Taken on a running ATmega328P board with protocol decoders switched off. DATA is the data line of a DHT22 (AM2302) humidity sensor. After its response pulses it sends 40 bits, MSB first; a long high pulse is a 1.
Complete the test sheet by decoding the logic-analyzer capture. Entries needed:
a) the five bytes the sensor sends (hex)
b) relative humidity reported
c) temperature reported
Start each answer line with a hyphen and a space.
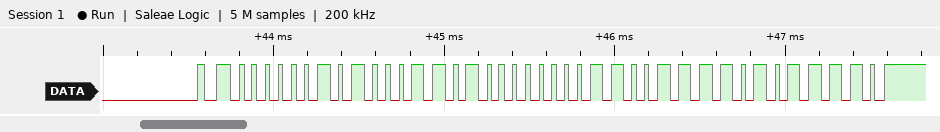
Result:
- 02 8D 00 CF 5E
- 65.3 %
- 20.7 °C
